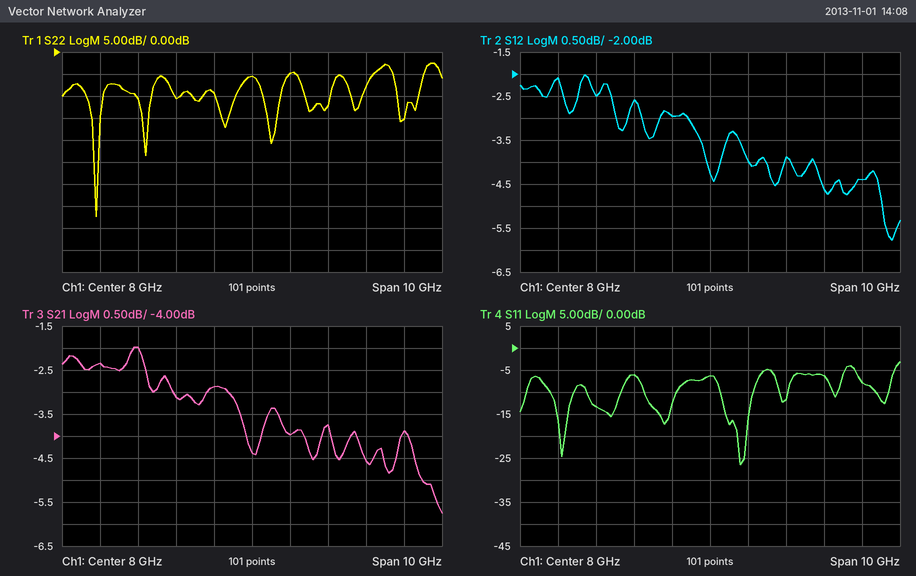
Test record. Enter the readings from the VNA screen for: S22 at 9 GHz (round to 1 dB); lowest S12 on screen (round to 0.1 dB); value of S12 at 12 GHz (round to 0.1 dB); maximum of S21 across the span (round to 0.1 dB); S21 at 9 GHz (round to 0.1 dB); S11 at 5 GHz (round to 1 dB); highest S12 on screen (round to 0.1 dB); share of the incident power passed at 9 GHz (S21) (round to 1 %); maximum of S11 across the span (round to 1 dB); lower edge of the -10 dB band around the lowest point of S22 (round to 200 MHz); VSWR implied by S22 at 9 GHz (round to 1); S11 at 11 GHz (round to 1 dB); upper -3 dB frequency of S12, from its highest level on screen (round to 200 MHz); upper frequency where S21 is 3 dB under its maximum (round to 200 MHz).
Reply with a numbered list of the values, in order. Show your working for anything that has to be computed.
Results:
1. -5 dB
2. -5.8 dB
3. -4.4 dB
4. -2.0 dB
5. -4.0 dB
6. -13 dB
7. -2.0 dB
8. 10^(-4/10) ≈ 40 %
9. -3 dB
10. 3.6 GHz
11. |Γ| = 10^(-5/20) = 0.5623; VSWR = (1 + 0.5623)/(1 − 0.5623) ≈ 4
12. -6 dB
13. 12.6 GHz
14. 12.4 GHz
